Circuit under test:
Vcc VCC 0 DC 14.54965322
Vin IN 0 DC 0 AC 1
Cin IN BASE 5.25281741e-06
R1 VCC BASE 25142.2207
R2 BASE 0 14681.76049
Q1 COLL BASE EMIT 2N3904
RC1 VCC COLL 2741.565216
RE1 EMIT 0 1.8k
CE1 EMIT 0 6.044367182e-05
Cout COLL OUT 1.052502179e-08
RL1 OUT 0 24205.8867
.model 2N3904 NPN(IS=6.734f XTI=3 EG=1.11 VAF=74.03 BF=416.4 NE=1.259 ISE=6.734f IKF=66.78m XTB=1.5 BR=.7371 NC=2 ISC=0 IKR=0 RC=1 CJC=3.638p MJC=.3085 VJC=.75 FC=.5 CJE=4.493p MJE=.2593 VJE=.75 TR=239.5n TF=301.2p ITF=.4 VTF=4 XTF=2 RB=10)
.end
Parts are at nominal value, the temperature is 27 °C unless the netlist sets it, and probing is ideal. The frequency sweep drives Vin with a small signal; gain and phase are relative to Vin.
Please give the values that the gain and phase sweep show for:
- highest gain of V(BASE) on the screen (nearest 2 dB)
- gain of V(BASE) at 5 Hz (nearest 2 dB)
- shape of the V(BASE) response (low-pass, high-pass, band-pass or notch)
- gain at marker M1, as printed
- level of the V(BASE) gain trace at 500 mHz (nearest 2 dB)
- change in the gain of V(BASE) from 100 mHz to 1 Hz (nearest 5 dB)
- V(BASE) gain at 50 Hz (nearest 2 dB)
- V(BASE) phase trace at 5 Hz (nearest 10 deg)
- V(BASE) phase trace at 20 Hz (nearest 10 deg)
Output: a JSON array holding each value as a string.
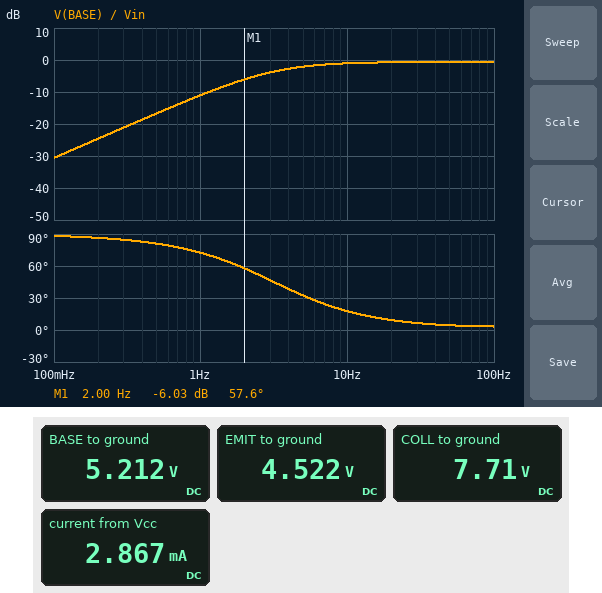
["0 dB", "-2 dB", "high-pass", "-6.03 dB", "-16 dB", "20 dB", "0 dB", "30 deg", "10 deg"]
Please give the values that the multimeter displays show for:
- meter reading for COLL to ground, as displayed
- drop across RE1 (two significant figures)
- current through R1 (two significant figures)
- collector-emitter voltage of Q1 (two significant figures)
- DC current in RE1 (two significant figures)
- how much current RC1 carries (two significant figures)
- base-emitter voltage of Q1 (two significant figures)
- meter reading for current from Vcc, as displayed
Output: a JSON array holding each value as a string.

["7.71 V", "4.5 V", "370 µA", "3.2 V", "2.5 mA", "2.5 mA", "690 mV", "2.867 mA"]
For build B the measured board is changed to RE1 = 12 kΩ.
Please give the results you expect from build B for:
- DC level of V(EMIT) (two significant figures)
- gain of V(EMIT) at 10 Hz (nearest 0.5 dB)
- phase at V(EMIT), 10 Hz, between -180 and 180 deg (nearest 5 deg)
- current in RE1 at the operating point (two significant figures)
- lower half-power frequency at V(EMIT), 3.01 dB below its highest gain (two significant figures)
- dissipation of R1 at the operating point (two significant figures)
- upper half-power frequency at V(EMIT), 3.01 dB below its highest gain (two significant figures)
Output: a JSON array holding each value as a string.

["4.7 V", "-1.5 dB", "5 deg", "390 µA", "2.7 Hz", "3.4 mW", "48 Hz"]
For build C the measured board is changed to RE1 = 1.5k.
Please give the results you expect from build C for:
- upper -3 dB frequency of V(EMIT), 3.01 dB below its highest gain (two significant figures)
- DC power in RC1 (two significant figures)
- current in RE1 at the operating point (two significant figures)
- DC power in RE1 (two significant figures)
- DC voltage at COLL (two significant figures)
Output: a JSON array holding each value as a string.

["290 Hz", "24 mW", "3.0 mA", "13 mW", "6.4 V"]
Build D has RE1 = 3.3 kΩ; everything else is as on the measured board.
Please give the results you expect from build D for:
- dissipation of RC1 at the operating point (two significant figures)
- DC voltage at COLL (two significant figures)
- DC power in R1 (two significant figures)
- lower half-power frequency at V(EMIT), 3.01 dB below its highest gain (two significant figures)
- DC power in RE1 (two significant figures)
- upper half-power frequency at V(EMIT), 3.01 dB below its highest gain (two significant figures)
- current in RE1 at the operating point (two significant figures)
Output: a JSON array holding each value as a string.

["5.3 mW", "11 V", "3.4 mW", "3.0 Hz", "6.4 mW", "150 Hz", "1.4 mA"]
